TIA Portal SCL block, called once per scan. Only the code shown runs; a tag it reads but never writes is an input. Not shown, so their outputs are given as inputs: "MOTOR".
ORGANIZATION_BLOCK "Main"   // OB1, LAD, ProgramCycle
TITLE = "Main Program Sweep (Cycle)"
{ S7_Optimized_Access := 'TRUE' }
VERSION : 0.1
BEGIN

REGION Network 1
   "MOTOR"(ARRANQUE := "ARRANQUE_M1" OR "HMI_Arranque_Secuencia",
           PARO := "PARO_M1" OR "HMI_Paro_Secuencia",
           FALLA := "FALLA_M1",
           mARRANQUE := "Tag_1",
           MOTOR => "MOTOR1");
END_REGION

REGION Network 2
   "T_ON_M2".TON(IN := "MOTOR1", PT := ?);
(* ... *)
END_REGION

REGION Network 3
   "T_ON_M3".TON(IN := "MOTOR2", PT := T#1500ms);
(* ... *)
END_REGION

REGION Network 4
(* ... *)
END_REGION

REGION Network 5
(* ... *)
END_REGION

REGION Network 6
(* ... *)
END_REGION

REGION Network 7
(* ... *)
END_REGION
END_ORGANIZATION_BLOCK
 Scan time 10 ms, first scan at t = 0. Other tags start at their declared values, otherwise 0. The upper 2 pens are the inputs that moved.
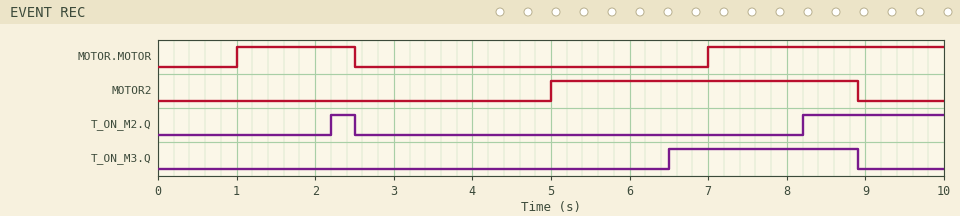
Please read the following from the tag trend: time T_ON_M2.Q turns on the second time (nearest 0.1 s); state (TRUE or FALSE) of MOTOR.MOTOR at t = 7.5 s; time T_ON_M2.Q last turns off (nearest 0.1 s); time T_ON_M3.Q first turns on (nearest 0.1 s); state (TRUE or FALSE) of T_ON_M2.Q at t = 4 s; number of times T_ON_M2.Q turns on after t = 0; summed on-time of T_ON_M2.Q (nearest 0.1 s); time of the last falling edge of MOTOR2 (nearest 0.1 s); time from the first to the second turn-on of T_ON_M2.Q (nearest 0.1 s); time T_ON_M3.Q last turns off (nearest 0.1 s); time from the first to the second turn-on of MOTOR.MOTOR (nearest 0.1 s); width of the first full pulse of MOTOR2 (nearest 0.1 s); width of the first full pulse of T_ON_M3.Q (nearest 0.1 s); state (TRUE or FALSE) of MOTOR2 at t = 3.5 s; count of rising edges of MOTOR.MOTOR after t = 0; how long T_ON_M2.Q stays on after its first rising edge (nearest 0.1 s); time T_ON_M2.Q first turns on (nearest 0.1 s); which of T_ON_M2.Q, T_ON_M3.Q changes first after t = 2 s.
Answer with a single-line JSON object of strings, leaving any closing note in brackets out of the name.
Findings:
{"time T_ON_M2.Q turns on the second time": "8.2 s", "state (TRUE or FALSE) of MOTOR.MOTOR at t = 7.5 s": "TRUE", "time T_ON_M2.Q last turns off": "2.5 s", "time T_ON_M3.Q first turns on": "6.5 s", "state (TRUE or FALSE) of T_ON_M2.Q at t = 4 s": "FALSE", "number of times T_ON_M2.Q turns on after t = 0": "2", "summed on-time of T_ON_M2.Q": "2.1 s", "time of the last falling edge of MOTOR2": "8.9 s", "time from the first to the second turn-on of T_ON_M2.Q": "6.0 s", "time T_ON_M3.Q last turns off": "8.9 s", "time from the first to the second turn-on of MOTOR.MOTOR": "6.0 s", "width of the first full pulse of MOTOR2": "3.9 s", "width of the first full pulse of T_ON_M3.Q": "2.4 s", "state (TRUE or FALSE) of MOTOR2 at t = 3.5 s": "FALSE", "count of rising edges of MOTOR.MOTOR after t = 0": "2", "how long T_ON_M2.Q stays on after its first rising edge": "0.3 s", "time T_ON_M2.Q first turns on": "2.2 s", "which of T_ON_M2.Q, T_ON_M3.Q changes first after t = 2 s": "T_ON_M2.Q"}
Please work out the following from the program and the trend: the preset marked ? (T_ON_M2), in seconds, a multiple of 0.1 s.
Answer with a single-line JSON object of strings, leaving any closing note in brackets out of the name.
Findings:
{"the preset marked ? (T_ON_M2), in seconds, a multiple of 0.1 s": "1.2 s"}
